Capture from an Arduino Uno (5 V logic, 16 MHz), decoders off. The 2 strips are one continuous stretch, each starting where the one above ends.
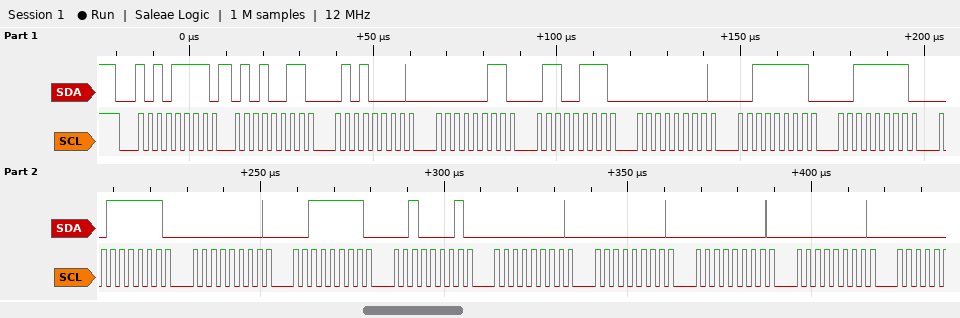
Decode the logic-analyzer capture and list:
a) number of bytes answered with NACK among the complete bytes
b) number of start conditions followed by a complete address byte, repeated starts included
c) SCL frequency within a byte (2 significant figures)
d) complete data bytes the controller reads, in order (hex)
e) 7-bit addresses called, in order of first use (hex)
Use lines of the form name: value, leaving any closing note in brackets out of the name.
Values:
number of bytes answered with NACK among the complete bytes: 0
number of start conditions followed by a complete address byte, repeated starts included: 1
SCL frequency within a byte: 400 kHz
complete data bytes the controller reads, in order: 53 50 03 67 00 3F 3F 3F 00 3F 21 00 00 00 00
7-bit addresses called, in order of first use: 0x57
